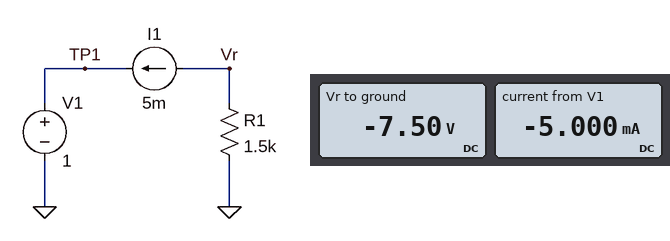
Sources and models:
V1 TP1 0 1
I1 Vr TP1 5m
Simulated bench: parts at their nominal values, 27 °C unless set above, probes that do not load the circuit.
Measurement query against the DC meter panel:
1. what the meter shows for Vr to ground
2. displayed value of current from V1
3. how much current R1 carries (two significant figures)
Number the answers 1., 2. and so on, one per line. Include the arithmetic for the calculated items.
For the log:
1. -7.50 V
2. -5.000 mA
3. (0 V - (-7.5 V)) / 1.5 kΩ = 5.0 mA
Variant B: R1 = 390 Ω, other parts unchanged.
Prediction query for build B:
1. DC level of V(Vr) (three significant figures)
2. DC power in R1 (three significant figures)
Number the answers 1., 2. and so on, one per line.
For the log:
1. -1.95 V
2. 9.75 mW
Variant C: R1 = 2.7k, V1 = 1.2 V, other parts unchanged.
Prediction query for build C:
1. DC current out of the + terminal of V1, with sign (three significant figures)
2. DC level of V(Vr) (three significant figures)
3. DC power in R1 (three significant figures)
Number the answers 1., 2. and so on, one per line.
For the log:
1. -5.00 mA
2. -13.5 V
3. 67.5 mW
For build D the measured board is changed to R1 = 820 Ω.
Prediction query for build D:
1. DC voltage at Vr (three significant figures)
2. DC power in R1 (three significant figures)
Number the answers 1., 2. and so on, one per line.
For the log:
1. -4.10 V
2. 20.5 mW
